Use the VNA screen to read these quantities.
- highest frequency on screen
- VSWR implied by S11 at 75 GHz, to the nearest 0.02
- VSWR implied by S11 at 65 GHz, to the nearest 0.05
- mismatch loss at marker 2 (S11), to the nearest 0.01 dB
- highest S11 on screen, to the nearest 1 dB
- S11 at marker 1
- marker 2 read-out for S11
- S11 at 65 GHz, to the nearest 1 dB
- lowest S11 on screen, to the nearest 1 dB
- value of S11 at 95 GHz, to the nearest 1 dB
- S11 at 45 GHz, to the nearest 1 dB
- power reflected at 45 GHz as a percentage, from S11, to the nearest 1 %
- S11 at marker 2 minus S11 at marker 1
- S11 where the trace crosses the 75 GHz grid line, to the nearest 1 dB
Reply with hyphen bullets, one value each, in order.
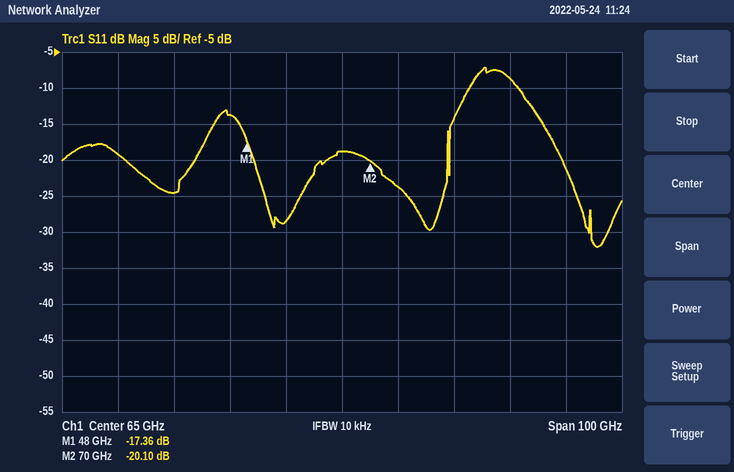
- 115 GHz
- 1.14
- 1.25
- 0.04 dB
- -7 dB
- -17.36 dB
- -20.10 dB
- -19 dB
- -32 dB
- -9 dB
- -14 dB
- 4 %
- -2.74 dB
- -24 dB
